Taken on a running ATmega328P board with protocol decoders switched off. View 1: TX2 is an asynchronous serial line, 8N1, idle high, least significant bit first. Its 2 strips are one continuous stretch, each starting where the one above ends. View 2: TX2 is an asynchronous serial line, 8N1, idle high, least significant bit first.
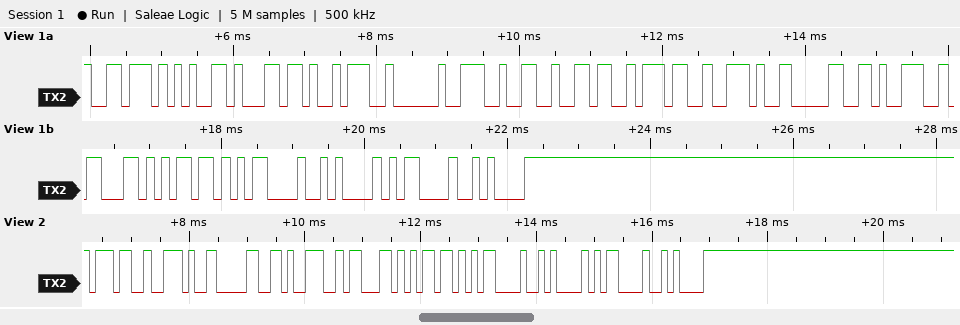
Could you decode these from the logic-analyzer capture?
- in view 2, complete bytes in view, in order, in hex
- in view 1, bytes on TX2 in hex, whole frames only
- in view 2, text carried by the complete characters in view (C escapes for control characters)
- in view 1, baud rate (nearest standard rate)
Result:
37 2E 30 39 63 6D 0D 0A 0D 0A
76 65 6C 3A 20 32 36 37 2E 30 39 63 6D 0D 0A 0D 0A
"7.09cm\r\n\r\n"
9600 baud
